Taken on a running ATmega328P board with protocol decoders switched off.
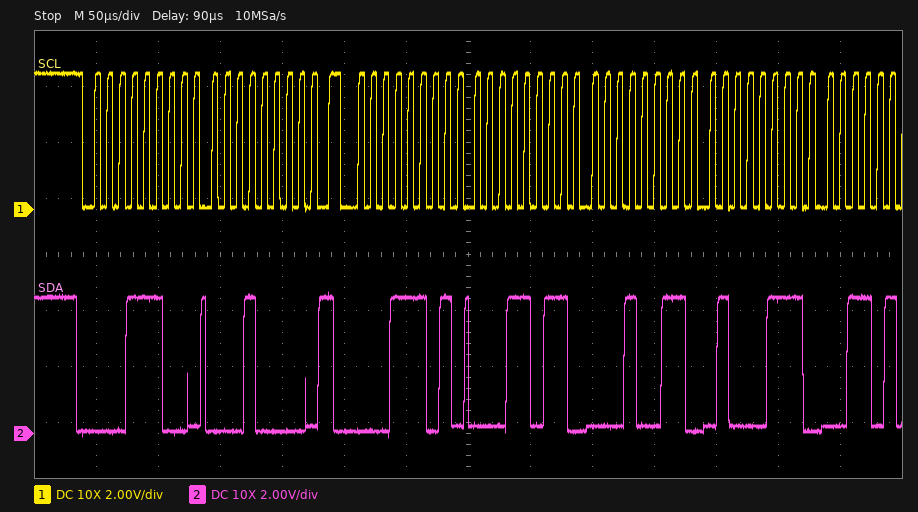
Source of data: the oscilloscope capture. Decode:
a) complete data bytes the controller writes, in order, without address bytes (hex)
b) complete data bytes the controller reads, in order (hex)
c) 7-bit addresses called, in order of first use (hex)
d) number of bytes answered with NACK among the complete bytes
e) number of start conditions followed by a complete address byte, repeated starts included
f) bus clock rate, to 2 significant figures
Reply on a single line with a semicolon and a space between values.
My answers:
10; 1B 13 47; 0x0E; 0; 2; 100 kHz
